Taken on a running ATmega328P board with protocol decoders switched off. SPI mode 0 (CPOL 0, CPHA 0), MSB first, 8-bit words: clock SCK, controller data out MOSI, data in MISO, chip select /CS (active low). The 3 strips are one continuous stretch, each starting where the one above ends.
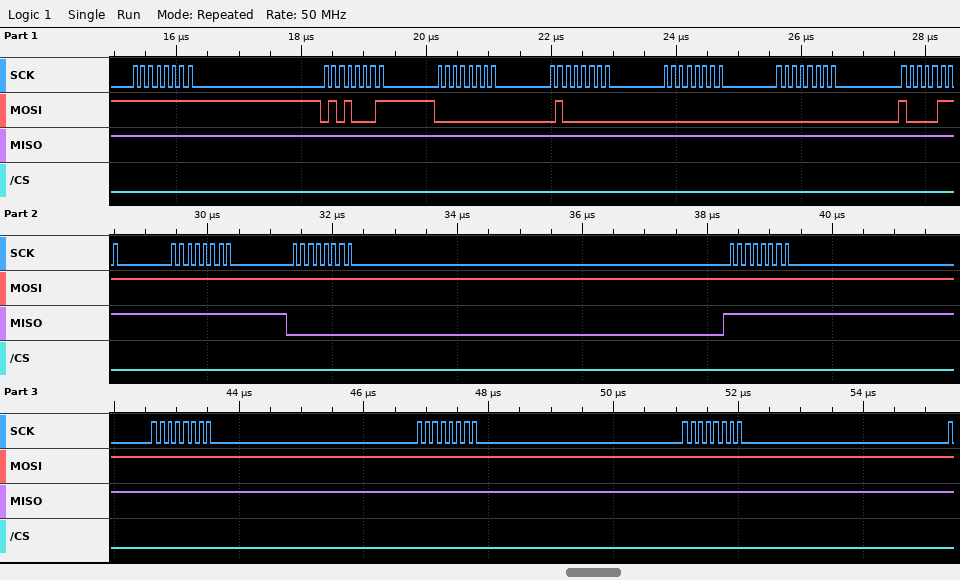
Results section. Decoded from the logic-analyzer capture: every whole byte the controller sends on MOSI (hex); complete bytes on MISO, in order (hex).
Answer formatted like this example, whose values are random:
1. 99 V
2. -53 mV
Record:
1. FF 51 00 40 00 00 87 FF FF FF FF FF FF
2. FF FF FF FF FF FF FF FF 00 FF FF FF FF
